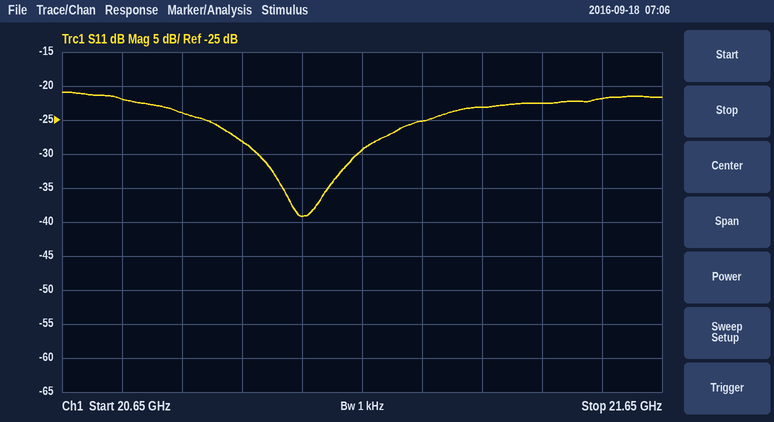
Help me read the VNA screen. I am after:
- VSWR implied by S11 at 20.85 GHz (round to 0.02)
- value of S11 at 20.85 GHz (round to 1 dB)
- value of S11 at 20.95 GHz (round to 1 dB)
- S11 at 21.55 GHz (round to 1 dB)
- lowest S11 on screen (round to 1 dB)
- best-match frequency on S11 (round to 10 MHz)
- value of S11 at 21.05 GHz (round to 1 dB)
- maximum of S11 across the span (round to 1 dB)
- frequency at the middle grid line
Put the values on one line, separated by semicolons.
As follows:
1.14; -24 dB; -28 dB; -22 dB; -39 dB; 21.05 GHz; -39 dB; -21 dB; 21.15 GHz
